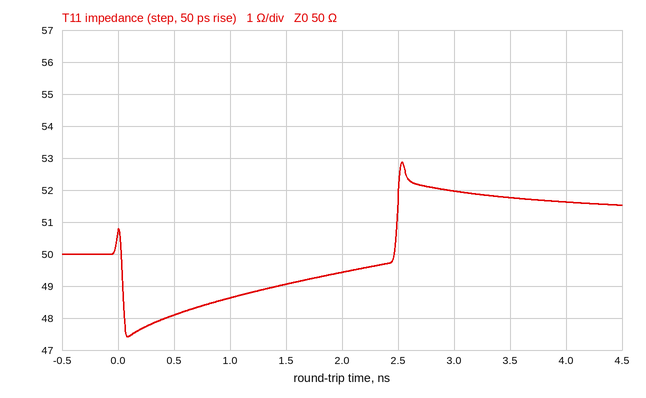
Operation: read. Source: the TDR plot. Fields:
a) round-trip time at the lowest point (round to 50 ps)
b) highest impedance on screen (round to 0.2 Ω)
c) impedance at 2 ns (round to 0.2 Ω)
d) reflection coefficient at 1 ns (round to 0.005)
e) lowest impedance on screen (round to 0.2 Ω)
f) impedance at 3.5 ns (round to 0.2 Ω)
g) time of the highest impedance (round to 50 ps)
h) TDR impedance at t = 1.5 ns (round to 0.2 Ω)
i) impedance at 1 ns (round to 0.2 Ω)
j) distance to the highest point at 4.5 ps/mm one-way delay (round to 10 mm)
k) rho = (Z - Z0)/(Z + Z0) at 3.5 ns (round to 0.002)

100 ps
52.8 Ω
49.4 Ω
-0.015
47.4 Ω
51.8 Ω
2.55 ns
49.0 Ω
48.6 Ω
280 mm
+0.018
